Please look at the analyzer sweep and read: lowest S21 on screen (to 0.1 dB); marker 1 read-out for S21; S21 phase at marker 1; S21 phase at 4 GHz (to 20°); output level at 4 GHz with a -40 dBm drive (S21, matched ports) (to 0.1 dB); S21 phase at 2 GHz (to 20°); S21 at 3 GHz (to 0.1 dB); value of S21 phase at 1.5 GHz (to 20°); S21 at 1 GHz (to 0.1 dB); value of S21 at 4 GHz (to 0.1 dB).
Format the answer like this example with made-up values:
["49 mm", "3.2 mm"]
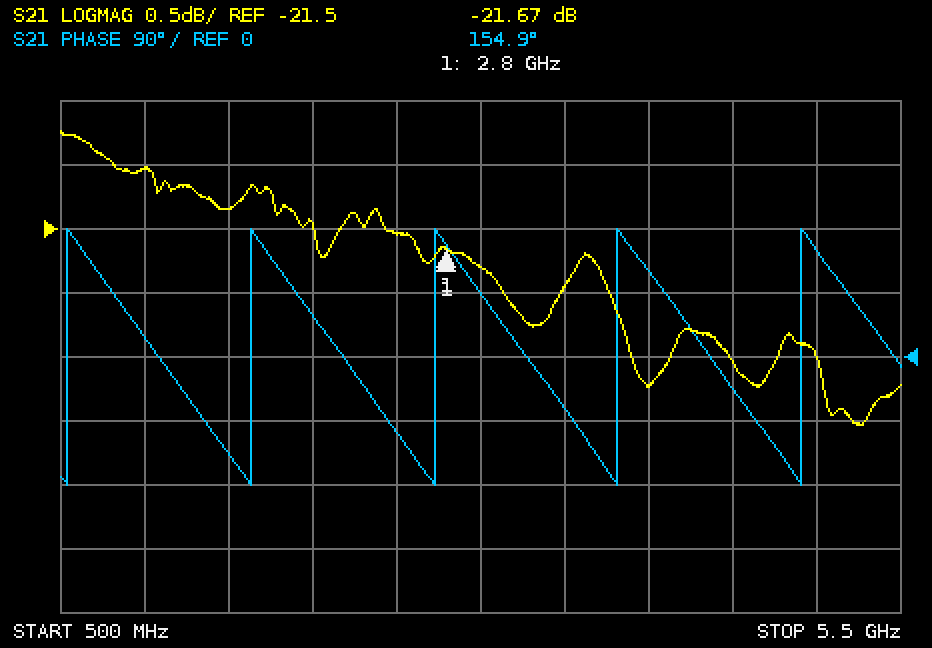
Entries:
["-23.0 dB", "-21.67 dB", "154.9°", "120°", "-62.7 dBm", "60°", "-21.8 dB", "-140°", "-21.0 dB", "-22.7 dB"]
